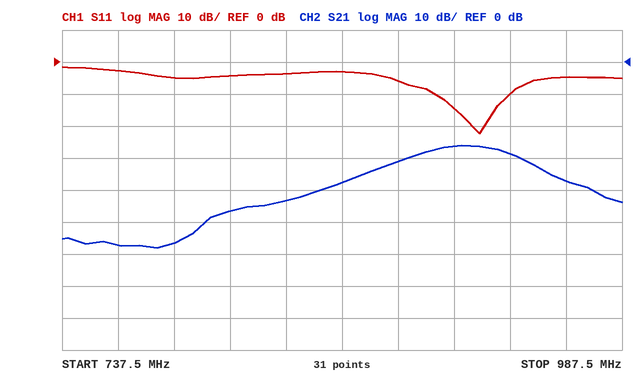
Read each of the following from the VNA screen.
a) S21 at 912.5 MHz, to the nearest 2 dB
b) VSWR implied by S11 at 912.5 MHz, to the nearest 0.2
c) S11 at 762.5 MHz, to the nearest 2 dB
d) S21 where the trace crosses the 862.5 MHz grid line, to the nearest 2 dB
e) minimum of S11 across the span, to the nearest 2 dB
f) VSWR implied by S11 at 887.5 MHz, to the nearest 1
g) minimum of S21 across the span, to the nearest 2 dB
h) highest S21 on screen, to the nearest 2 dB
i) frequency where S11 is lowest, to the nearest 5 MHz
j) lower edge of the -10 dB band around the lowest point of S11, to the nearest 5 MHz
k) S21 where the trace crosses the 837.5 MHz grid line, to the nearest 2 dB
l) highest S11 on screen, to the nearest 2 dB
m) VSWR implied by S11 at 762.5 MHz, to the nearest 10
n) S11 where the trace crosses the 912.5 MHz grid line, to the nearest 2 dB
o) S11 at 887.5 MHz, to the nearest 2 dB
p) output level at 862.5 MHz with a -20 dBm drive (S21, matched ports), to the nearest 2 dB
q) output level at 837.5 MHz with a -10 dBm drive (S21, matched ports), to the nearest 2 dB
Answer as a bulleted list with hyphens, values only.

- -26 dB
- 1.4
- -2 dB
- -38 dB
- -22 dB
- 3
- -58 dB
- -26 dB
- 925 MHz
- 905 MHz
- -44 dB
- -2 dB
- 10
- -14 dB
- -6 dB
- -58 dBm
- -54 dBm
